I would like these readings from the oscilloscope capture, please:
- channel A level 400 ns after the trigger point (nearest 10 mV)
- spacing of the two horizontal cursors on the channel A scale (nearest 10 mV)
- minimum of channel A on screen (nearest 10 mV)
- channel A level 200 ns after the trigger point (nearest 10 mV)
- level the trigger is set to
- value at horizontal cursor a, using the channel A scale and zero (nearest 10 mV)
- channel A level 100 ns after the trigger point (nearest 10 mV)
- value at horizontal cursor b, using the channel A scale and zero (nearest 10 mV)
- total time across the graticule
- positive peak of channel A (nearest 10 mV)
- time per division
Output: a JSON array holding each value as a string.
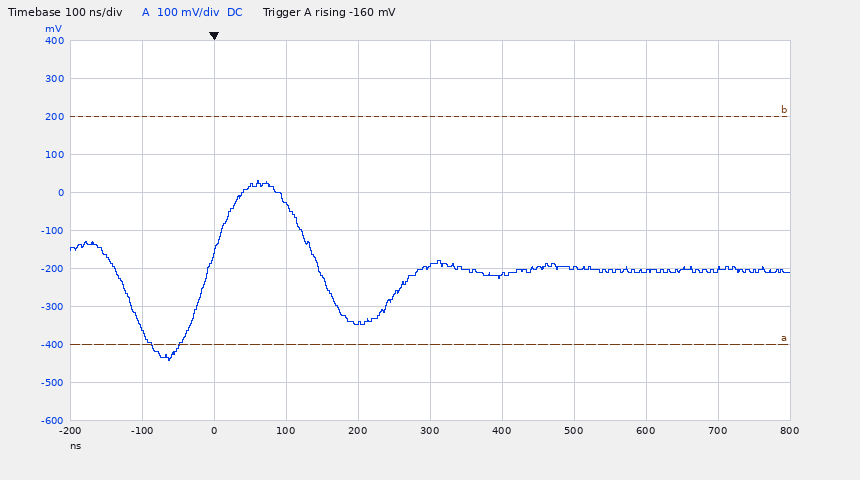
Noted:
["-220 mV", "600 mV", "-440 mV", "-340 mV", "-160 mV", "-400 mV", "-30 mV", "200 mV", "1 µs", "30 mV", "100 ns"]
